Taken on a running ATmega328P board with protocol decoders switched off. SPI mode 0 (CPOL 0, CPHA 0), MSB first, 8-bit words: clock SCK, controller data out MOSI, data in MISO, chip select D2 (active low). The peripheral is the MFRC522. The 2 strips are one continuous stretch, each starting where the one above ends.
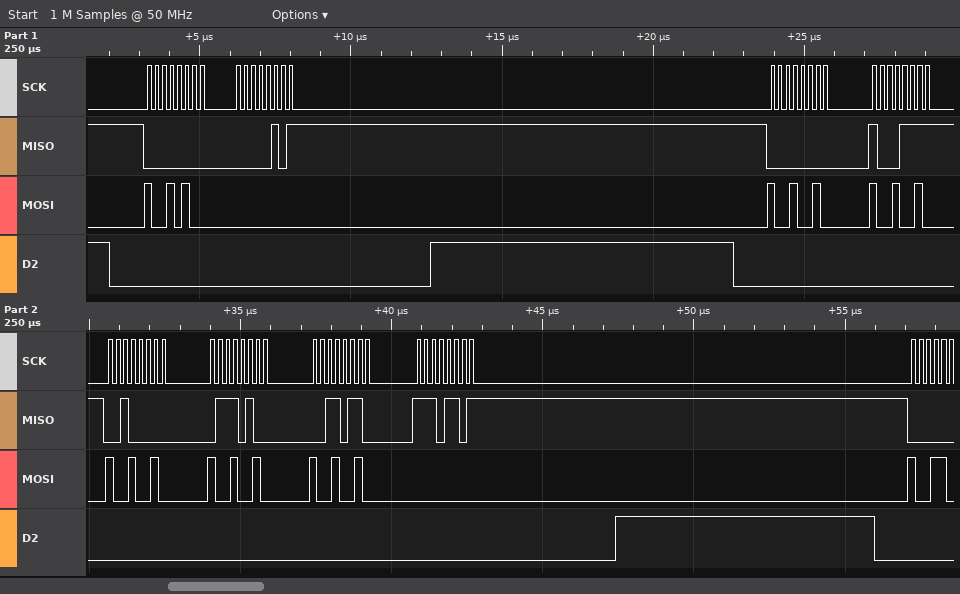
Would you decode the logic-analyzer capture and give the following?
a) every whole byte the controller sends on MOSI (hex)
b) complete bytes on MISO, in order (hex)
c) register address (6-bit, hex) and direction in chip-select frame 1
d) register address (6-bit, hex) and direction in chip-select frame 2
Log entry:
0x94 0x00 0x92 0x92 0x92 0x92 0x92 0x00
0x00 0x05 0x00 0x8F 0x20 0x74 0x36 0xED
0x0A read
0x09 read
